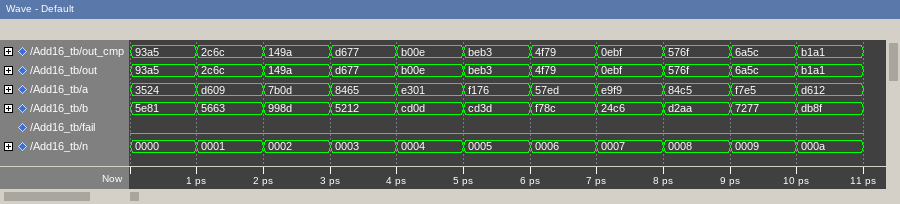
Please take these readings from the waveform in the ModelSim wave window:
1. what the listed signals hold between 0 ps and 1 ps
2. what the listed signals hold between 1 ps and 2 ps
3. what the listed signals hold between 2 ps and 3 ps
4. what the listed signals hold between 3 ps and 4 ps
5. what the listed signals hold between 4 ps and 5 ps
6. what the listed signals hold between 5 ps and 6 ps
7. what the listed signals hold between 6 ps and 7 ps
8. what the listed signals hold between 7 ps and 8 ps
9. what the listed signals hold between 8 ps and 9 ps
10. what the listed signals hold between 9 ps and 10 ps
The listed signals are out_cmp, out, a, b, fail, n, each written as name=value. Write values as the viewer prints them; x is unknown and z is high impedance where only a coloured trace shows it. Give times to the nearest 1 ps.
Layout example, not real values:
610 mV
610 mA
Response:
out_cmp=93a5, out=93a5, a=3524, b=5e81, fail=0, n=0000
out_cmp=2c6c, out=2c6c, a=d609, b=5663, fail=0, n=0001
out_cmp=149a, out=149a, a=7b0d, b=998d, fail=0, n=0002
out_cmp=d677, out=d677, a=8465, b=5212, fail=0, n=0003
out_cmp=b00e, out=b00e, a=e301, b=cd0d, fail=0, n=0004
out_cmp=beb3, out=beb3, a=f176, b=cd3d, fail=0, n=0005
out_cmp=4f79, out=4f79, a=57ed, b=f78c, fail=0, n=0006
out_cmp=0ebf, out=0ebf, a=e9f9, b=24c6, fail=0, n=0007
out_cmp=576f, out=576f, a=84c5, b=d2aa, fail=0, n=0008
out_cmp=6a5c, out=6a5c, a=f7e5, b=7277, fail=0, n=0009
